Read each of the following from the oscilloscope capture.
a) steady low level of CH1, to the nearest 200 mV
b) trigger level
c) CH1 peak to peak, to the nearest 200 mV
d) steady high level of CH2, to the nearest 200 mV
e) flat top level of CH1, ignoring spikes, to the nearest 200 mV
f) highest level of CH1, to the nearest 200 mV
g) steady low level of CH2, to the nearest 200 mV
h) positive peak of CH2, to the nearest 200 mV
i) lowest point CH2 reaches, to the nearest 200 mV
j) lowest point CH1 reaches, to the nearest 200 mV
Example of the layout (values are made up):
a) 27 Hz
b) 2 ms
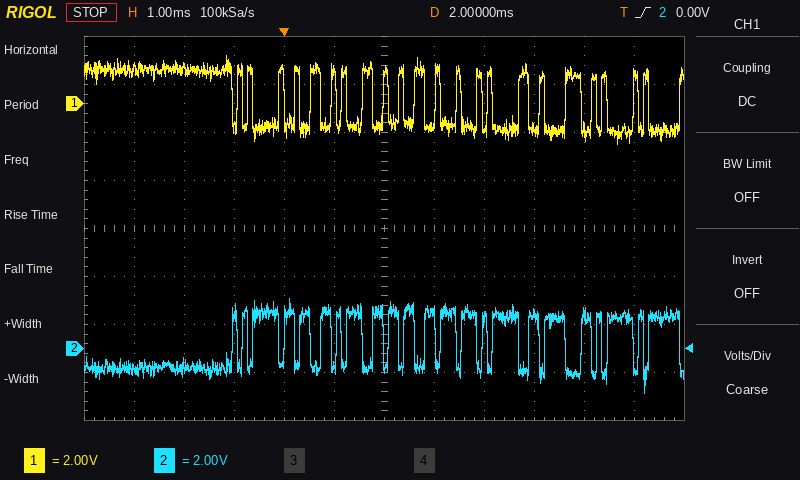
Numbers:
a) -1.0 V
b) 0.00 V
c) 3.6 V
d) 1.4 V
e) 1.4 V
f) 2.0 V
g) -800 mV
h) 2.0 V
i) -1.8 V
j) -1.6 V
